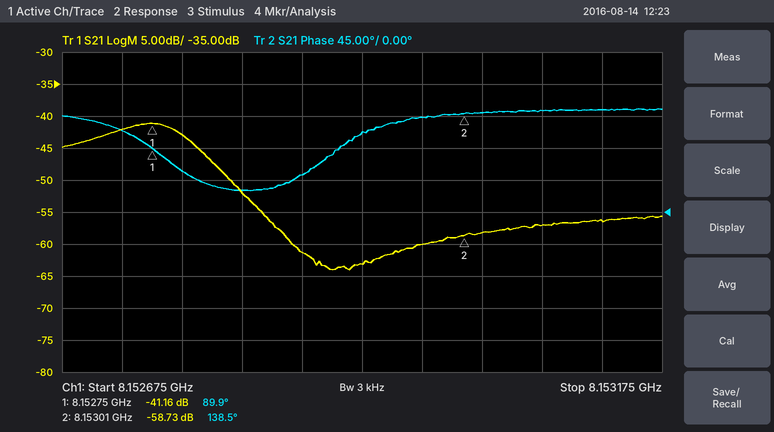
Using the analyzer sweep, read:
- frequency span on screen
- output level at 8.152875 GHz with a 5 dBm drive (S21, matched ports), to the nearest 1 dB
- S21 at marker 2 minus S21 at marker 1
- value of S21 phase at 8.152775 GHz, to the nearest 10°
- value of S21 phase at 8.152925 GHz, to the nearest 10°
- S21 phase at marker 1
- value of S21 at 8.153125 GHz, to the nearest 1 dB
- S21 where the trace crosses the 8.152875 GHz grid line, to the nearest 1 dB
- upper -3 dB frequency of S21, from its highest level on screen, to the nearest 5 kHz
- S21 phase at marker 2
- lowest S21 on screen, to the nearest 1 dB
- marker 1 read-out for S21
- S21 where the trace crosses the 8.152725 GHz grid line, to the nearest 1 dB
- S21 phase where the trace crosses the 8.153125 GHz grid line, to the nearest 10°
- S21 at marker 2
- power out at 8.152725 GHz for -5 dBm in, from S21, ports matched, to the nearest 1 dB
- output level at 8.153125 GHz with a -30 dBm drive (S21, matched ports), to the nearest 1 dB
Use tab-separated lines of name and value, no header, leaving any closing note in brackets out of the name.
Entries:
frequency span on screen	500 kHz
output level at 8.152875 GHz with a 5 dBm drive (S21, matched ports), to the nearest 1 dB	-56 dBm
S21 at marker 2 minus S21 at marker 1	-17.57 dB
value of S21 phase at 8.152775 GHz, to the nearest 10°	60°
value of S21 phase at 8.152925 GHz, to the nearest 10°	110°
S21 phase at marker 1	89.9°
value of S21 at 8.153125 GHz, to the nearest 1 dB	-56 dB
S21 where the trace crosses the 8.152875 GHz grid line, to the nearest 1 dB	-61 dB
upper -3 dB frequency of S21, from its highest level on screen, to the nearest 5 kHz	8.152785 GHz
S21 phase at marker 2	138.5°
lowest S21 on screen, to the nearest 1 dB	-64 dB
marker 1 read-out for S21	-41.16 dB
S21 where the trace crosses the 8.152725 GHz grid line, to the nearest 1 dB	-42 dB
S21 phase where the trace crosses the 8.153125 GHz grid line, to the nearest 10°	140°
S21 at marker 2	-58.73 dB
power out at 8.152725 GHz for -5 dBm in, from S21, ports matched, to the nearest 1 dB	-47 dBm
output level at 8.153125 GHz with a -30 dBm drive (S21, matched ports), to the nearest 1 dB	-86 dBm
